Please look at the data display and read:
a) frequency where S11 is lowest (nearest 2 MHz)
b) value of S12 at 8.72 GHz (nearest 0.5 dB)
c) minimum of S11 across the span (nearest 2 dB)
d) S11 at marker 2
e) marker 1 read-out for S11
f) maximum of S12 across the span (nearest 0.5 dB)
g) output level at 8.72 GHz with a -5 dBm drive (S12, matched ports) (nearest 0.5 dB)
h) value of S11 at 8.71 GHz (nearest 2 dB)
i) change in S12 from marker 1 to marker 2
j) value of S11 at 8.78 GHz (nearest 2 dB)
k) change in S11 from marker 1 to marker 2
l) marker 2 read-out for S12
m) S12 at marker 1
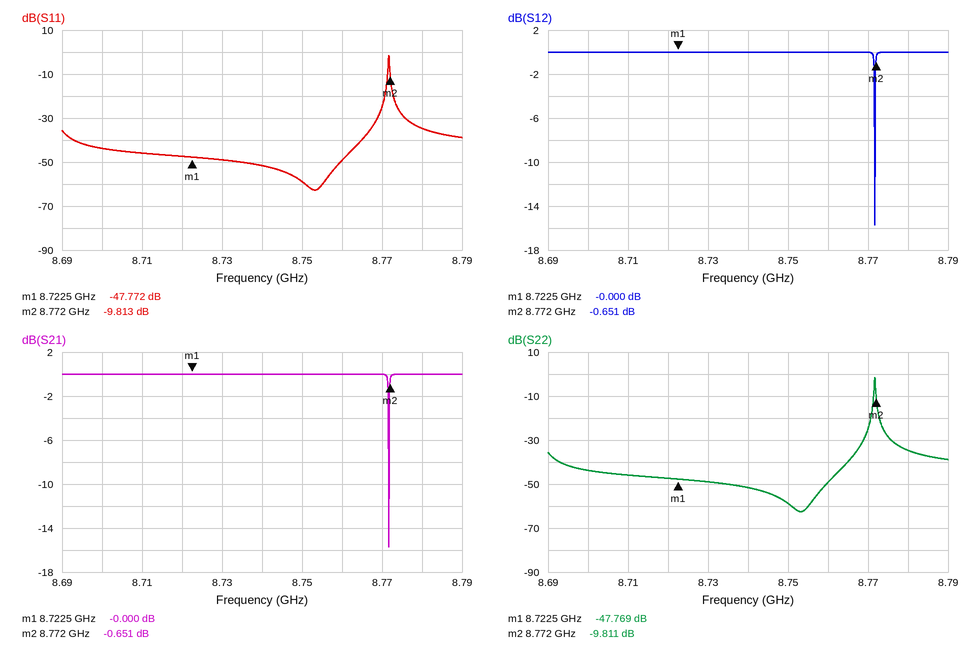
8.754 GHz
0.0 dB
-62 dB
-9.813 dB
-47.772 dB
0.0 dB
-5.0 dBm
-46 dB
-0.651 dB
-34 dB
37.959 dB
-0.651 dB
-0.000 dB
